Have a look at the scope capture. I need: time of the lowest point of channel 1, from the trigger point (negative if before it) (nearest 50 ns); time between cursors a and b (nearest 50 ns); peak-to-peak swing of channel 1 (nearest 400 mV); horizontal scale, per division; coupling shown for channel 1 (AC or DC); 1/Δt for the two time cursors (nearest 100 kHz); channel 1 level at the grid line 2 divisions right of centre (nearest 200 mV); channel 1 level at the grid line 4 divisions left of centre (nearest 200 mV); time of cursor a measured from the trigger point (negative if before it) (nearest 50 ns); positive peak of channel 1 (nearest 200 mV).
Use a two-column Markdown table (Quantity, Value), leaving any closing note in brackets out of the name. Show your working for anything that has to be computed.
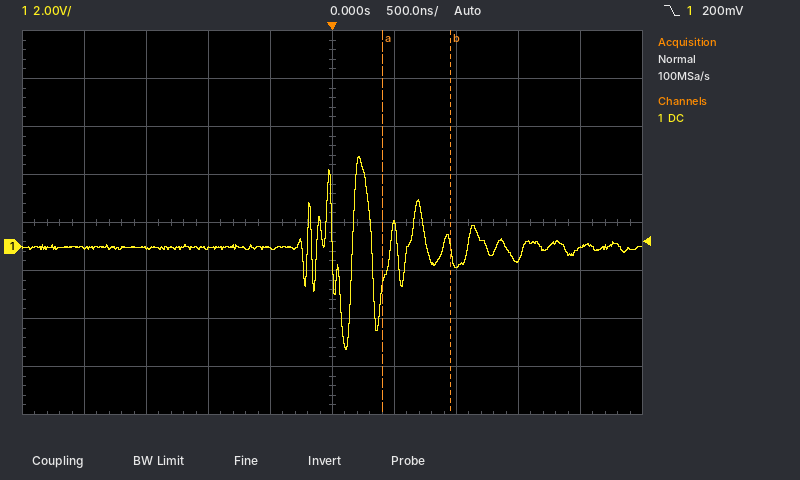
| Quantity | Value |
|---|---|
| time of the lowest point of channel 1, from the trigger point (negative if before it) | +100 ns |
| time between cursors a and b | 550 ns |
| peak-to-peak swing of channel 1 | 8.0 V |
| horizontal scale, per division | 500 ns |
| coupling shown for channel 1 | DC |
| 1/Δt for the two time cursors | 1 / 550 ns ≈ 1.8 MHz |
| channel 1 level at the grid line 2 divisions right of centre | -800 mV |
| channel 1 level at the grid line 4 divisions left of centre | 0.0 V |
| time of cursor a measured from the trigger point (negative if before it) | +400 ns |
| positive peak of channel 1 | 3.8 V |
